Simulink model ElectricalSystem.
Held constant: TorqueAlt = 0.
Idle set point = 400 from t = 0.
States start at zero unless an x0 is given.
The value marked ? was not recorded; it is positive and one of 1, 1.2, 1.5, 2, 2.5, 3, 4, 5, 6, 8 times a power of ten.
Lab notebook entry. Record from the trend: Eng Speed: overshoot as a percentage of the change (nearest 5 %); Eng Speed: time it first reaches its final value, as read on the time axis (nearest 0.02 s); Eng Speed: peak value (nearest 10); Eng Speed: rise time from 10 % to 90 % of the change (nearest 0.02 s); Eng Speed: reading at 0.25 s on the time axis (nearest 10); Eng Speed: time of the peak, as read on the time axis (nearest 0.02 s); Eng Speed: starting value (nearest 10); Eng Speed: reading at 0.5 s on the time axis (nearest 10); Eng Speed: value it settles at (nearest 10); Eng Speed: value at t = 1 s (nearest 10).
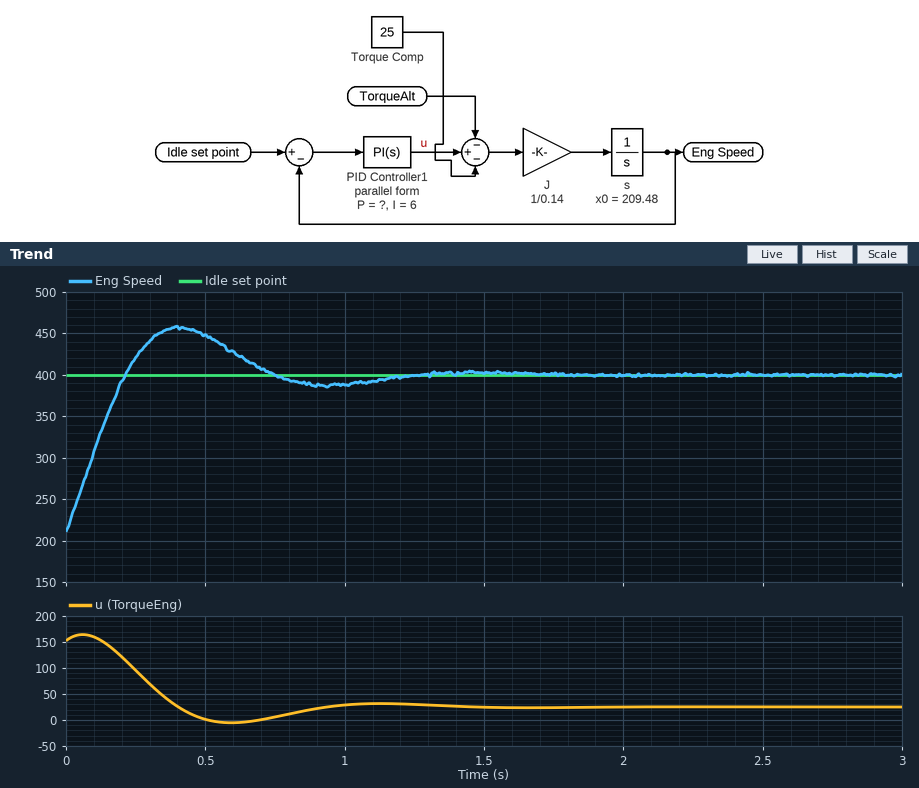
30 %
0.22 s
460
0.16 s
420
0.40 s
210
450
400
390
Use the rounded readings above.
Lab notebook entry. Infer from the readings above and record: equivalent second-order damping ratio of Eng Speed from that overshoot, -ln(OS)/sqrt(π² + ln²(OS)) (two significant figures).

0.36
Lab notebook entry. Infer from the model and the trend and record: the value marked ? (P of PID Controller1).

0.8
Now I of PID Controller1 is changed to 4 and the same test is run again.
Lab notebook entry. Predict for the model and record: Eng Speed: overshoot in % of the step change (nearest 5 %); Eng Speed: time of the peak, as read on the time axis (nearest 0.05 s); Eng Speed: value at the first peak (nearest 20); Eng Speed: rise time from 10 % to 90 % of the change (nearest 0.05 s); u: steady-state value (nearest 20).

25 %
0.50 s
440
0.20 s
20
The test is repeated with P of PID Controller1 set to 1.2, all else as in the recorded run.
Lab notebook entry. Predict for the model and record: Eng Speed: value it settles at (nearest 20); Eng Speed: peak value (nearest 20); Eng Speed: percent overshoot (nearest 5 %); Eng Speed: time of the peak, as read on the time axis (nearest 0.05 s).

400
440
20 %
0.35 s
